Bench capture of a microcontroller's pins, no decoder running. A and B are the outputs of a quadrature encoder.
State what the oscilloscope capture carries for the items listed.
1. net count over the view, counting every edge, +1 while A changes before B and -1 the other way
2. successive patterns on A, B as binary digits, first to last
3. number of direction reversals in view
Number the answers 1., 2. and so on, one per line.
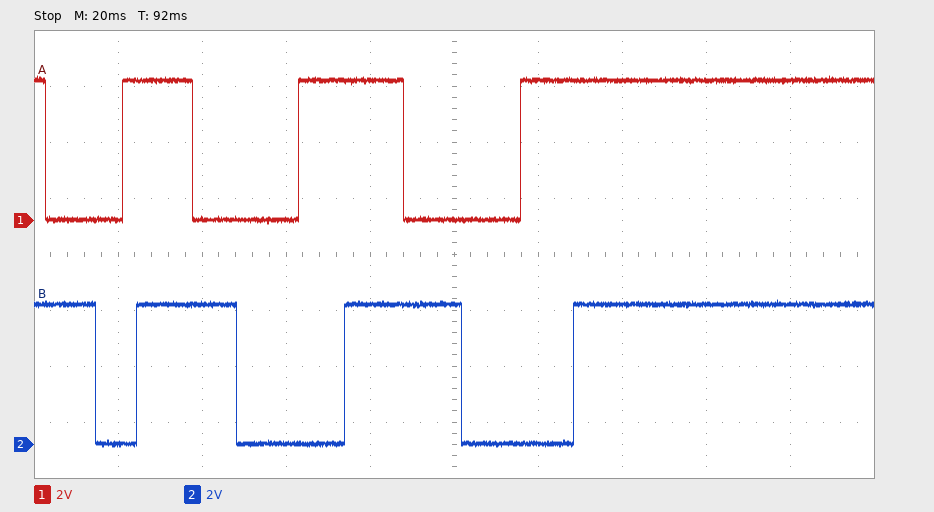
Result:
1. +12
2. 11 01 00 10 11 01 00 10 11 01 00 10 11
3. 0
